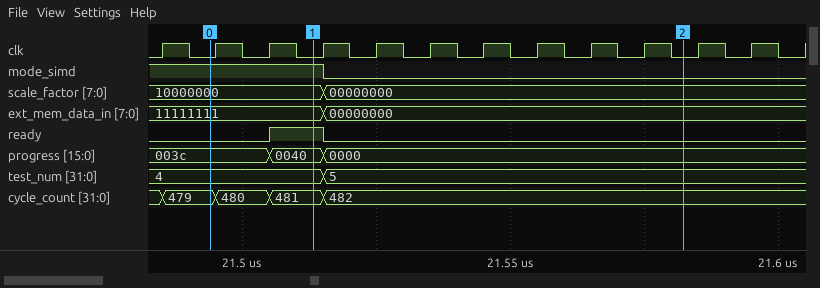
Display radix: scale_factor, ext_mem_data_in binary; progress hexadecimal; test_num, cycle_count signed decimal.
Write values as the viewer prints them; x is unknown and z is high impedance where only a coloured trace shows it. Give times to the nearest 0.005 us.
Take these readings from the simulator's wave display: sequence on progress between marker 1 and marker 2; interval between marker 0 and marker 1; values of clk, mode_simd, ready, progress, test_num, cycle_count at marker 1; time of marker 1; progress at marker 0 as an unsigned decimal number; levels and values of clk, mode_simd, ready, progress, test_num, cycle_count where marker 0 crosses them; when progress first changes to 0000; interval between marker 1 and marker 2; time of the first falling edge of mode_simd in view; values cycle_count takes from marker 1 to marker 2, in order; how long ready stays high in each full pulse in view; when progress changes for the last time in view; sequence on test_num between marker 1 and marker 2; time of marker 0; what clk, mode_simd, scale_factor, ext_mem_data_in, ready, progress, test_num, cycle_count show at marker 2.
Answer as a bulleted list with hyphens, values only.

- 0040, 0000
- 0.02 us
- clk=0, mode_simd=1, ready=1, progress=0040, test_num=4, cycle_count=481
- 21.515 us
- 60
- clk=0, mode_simd=1, ready=0, progress=003c, test_num=4, cycle_count=479
- 21.515 us
- 0.07 us
- 21.515 us
- 481, 482
- 0.01 us
- 21.515 us
- 4, 5
- 21.495 us
- clk=0, mode_simd=0, scale_factor=00000000, ext_mem_data_in=00000000, ready=0, progress=0000, test_num=5, cycle_count=482
